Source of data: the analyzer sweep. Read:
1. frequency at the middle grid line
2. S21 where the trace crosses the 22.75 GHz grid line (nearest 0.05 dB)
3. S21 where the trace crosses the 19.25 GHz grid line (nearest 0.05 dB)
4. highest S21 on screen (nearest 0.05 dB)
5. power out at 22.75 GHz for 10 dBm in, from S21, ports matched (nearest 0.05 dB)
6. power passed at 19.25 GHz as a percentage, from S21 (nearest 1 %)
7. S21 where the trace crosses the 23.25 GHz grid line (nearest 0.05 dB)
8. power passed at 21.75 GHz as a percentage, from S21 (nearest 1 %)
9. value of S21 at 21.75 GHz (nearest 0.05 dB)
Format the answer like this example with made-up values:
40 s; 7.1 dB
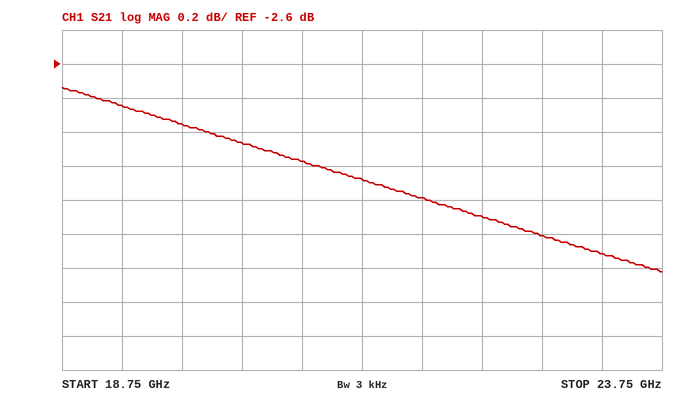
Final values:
21.25 GHz; -3.60 dB; -2.85 dB; -2.75 dB; 6.40 dBm; 52 %; -3.70 dB; 46 %; -3.40 dB
